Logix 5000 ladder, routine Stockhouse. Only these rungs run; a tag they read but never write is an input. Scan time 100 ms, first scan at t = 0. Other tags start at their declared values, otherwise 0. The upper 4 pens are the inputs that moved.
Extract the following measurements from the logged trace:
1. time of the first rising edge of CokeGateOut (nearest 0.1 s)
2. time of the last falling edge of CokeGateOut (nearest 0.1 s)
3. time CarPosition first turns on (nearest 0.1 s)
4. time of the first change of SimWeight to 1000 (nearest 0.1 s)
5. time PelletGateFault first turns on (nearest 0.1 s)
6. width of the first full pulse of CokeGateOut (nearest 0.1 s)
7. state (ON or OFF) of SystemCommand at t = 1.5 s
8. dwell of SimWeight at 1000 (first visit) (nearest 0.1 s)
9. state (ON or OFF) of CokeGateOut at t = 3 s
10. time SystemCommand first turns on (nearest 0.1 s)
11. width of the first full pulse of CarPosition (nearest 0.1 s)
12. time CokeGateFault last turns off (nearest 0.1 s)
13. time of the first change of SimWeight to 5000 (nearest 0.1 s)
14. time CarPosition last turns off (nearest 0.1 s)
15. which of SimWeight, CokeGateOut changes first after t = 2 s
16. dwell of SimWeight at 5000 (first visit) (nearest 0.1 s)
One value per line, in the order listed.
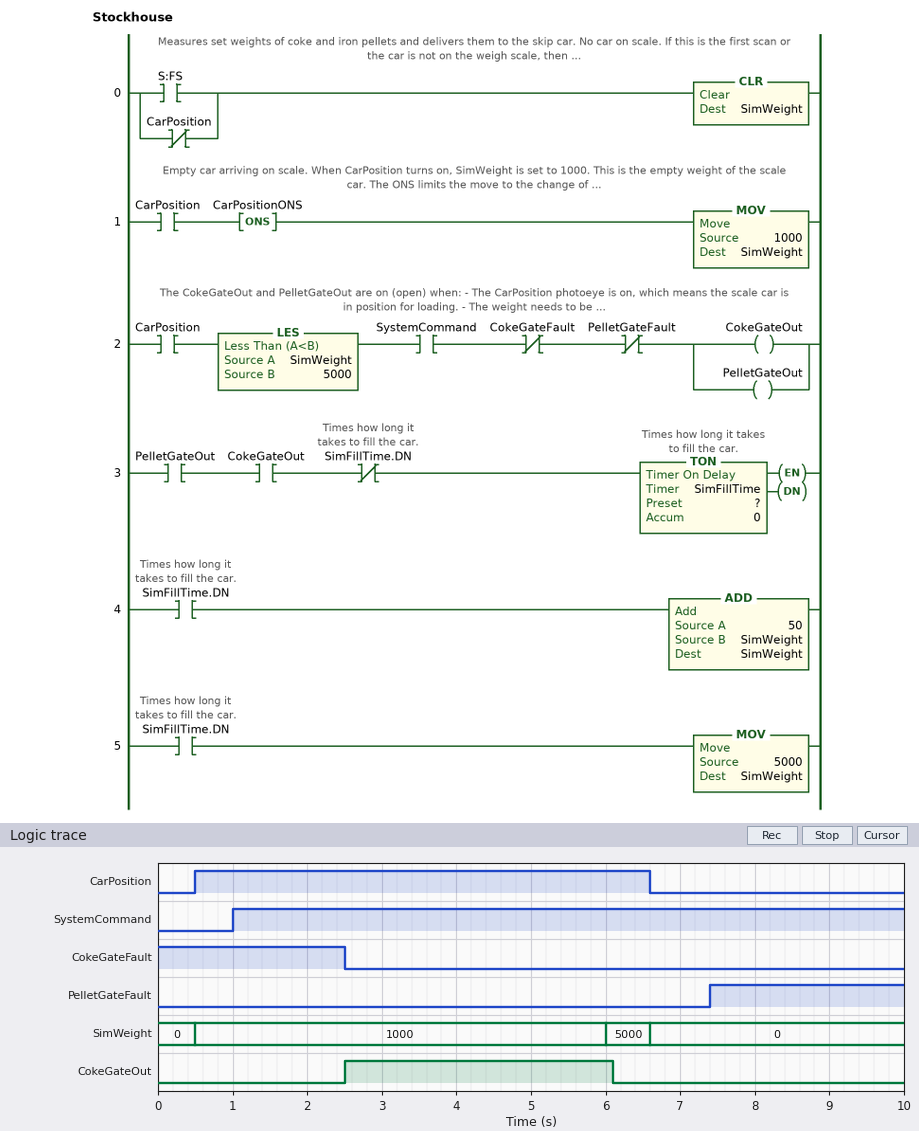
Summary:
2.5 s
6.1 s
0.5 s
0.5 s
7.4 s
3.6 s
ON
5.5 s
ON
1.0 s
6.1 s
2.5 s
6.0 s
6.6 s
CokeGateOut
0.6 s
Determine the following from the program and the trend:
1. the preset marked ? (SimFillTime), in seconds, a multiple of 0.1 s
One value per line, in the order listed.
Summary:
3.5 s
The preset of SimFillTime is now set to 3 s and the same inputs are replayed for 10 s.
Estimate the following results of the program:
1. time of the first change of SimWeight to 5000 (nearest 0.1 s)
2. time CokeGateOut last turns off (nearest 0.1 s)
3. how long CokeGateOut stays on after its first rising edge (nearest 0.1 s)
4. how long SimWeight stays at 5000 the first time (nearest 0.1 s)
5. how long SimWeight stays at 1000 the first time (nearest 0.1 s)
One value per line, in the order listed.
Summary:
5.5 s
5.6 s
3.1 s
1.1 s
5.0 s
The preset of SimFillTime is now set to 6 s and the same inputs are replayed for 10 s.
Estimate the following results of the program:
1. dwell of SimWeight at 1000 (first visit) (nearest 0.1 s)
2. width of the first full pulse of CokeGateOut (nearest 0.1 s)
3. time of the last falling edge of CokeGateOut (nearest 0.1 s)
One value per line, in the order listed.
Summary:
6.1 s
4.1 s
6.6 s
